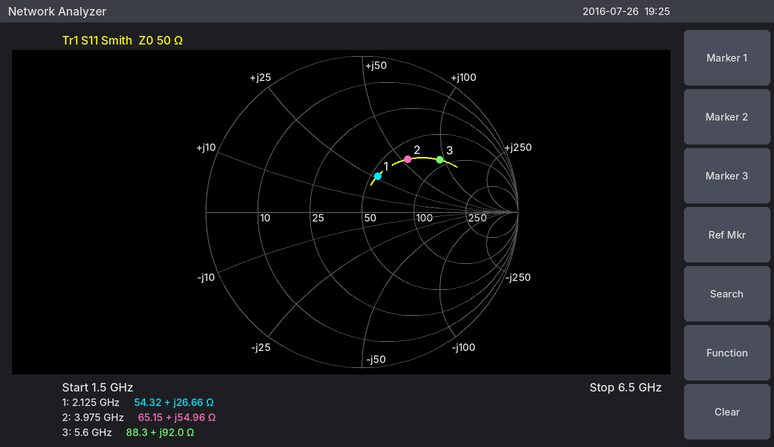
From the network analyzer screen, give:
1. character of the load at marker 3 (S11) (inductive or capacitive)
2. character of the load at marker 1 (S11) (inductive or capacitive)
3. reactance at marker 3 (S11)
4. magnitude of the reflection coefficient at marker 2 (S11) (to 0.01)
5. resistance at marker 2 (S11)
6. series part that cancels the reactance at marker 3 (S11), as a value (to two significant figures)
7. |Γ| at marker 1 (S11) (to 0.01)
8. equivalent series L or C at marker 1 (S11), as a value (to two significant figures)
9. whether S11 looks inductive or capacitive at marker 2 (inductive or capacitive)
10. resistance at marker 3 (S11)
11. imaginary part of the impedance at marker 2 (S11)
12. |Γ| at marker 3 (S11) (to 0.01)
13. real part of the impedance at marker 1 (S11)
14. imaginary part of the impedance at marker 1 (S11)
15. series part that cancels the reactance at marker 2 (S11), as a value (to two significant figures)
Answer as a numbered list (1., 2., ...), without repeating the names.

1. inductive
2. inductive
3. +92.0 Ω
4. 0.45
5. 65.15 Ω
6. 310 fF
7. 0.25
8. 2.0 nH
9. inductive
10. 88.3 Ω
11. +54.96 Ω
12. 0.60
13. 54.32 Ω
14. +26.66 Ω
15. 730 fF
